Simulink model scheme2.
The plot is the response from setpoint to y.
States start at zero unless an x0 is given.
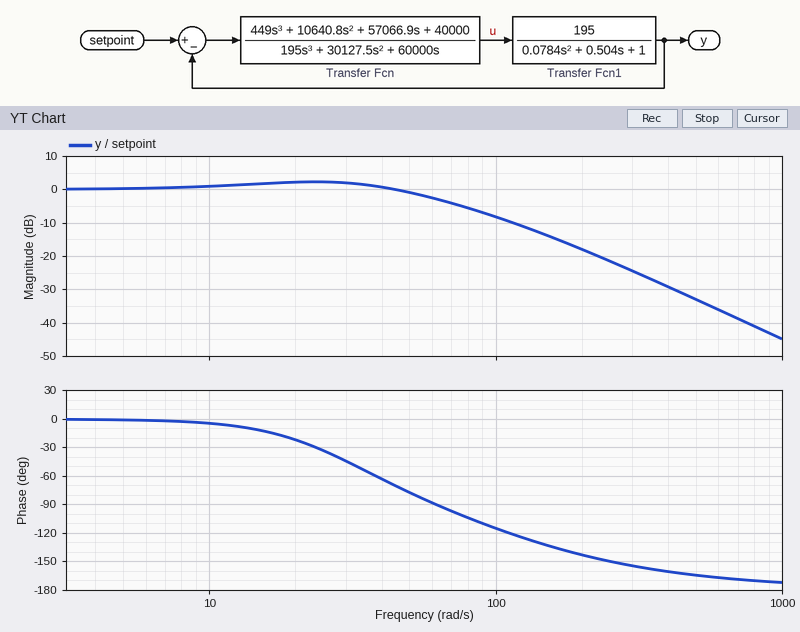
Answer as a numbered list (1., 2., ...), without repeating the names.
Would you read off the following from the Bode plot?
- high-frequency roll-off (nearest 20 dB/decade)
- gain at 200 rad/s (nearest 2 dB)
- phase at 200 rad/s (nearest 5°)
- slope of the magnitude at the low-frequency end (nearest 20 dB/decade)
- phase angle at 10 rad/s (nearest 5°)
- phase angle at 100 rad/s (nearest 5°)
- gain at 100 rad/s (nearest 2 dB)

1. -40 dB/decade
2. -18 dB
3. -145°
4. 0 dB/decade
5. -5°
6. -115°
7. -8 dB
